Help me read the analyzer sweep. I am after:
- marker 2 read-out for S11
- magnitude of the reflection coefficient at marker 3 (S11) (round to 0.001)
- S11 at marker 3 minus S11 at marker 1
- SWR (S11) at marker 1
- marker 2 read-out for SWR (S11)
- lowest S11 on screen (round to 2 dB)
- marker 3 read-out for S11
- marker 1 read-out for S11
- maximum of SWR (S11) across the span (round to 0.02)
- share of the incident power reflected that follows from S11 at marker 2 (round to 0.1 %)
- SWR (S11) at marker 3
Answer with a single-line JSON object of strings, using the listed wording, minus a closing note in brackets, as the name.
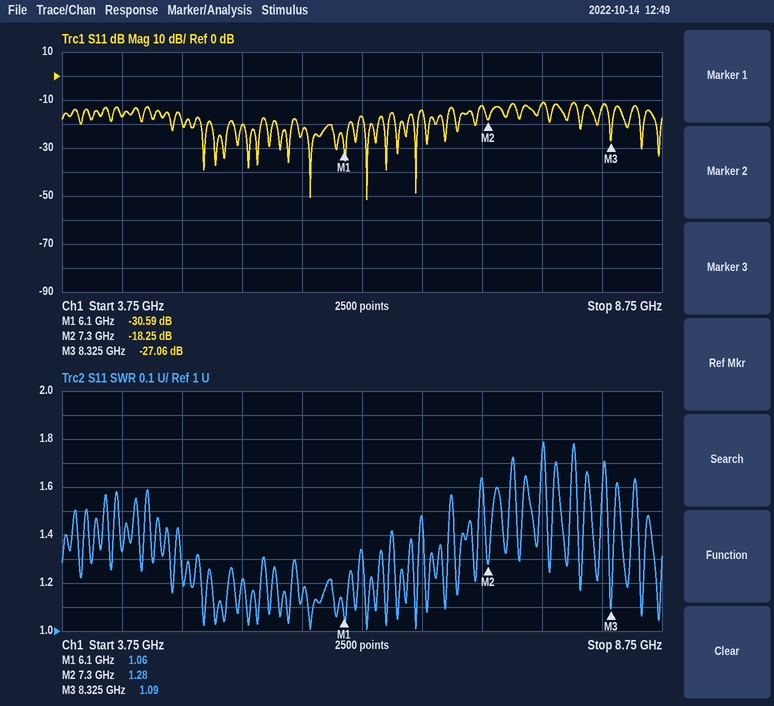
{"marker 2 read-out for S11": "-18.25 dB", "magnitude of the reflection coefficient at marker 3 (S11)": "0.044", "S11 at marker 3 minus S11 at marker 1": "3.53 dB", "SWR (S11) at marker 1": "1.06", "marker 2 read-out for SWR": "1.28", "lowest S11 on screen": "-52 dB", "marker 3 read-out for S11": "-27.06 dB", "marker 1 read-out for S11": "-30.59 dB", "maximum of SWR (S11) across the span": "1.78", "share of the incident power reflected that follows from S11 at marker 2": "1.5 %", "SWR (S11) at marker 3": "1.09"}
